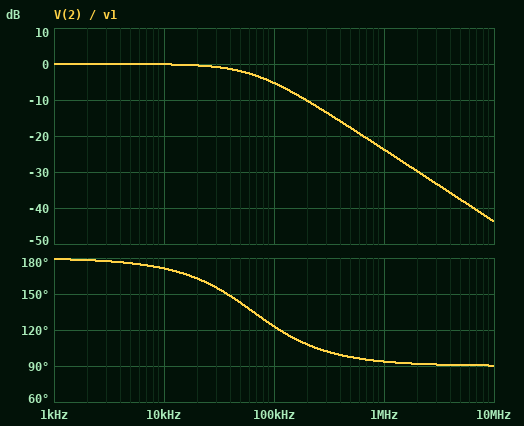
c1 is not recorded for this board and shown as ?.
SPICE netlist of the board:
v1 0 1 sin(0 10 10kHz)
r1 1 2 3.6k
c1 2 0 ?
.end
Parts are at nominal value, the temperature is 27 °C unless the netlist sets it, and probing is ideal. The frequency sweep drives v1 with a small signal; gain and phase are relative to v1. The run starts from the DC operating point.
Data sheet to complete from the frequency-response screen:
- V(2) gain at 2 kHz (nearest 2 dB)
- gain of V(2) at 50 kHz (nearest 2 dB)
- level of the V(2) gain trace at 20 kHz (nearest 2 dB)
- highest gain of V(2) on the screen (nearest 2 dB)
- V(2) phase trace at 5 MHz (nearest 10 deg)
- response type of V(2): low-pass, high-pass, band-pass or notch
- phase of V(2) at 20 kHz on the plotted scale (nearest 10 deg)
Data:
0 dB
-2 dB
0 dB
0 dB
90 deg
low-pass
160 deg
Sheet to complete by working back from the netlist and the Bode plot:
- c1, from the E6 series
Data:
680 pF
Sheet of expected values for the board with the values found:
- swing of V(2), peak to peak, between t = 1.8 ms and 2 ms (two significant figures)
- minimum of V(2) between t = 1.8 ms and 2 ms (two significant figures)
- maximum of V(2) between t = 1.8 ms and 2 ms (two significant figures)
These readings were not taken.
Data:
20 V
-9.9 V
9.9 V
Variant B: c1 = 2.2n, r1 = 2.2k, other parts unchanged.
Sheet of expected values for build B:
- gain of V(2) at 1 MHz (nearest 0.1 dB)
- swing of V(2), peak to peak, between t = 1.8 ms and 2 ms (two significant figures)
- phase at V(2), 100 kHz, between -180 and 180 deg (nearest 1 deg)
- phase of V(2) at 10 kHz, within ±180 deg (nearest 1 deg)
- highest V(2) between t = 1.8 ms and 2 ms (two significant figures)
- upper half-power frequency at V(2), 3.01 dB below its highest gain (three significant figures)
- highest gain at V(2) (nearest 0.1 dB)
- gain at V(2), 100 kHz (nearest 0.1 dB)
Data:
-29.7 dB
19 V
108 deg
163 deg
9.6 V
32.9 kHz
0 dB
-10.1 dB
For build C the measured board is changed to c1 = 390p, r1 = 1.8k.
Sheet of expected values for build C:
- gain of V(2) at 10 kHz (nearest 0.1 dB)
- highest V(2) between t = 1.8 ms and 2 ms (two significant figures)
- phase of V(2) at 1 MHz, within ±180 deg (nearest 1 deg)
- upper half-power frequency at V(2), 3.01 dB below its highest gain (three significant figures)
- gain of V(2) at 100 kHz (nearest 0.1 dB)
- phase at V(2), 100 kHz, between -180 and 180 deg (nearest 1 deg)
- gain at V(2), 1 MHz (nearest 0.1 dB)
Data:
0 dB
10 V
103 deg
227 kHz
-0.8 dB
156 deg
-13.1 dB
